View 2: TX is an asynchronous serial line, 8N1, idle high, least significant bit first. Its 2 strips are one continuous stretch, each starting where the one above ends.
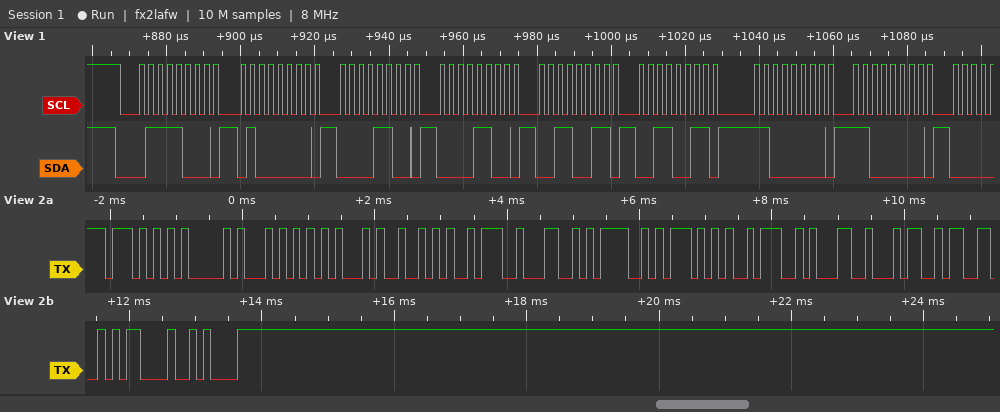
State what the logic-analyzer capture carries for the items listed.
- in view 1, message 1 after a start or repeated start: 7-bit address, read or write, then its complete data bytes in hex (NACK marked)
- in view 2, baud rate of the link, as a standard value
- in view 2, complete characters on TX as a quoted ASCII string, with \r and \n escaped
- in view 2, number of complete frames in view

0x3C write: 40 0C 0C 33 33 C0 C0
9600 baud
"WATER:LOW:143\r\n"
15
